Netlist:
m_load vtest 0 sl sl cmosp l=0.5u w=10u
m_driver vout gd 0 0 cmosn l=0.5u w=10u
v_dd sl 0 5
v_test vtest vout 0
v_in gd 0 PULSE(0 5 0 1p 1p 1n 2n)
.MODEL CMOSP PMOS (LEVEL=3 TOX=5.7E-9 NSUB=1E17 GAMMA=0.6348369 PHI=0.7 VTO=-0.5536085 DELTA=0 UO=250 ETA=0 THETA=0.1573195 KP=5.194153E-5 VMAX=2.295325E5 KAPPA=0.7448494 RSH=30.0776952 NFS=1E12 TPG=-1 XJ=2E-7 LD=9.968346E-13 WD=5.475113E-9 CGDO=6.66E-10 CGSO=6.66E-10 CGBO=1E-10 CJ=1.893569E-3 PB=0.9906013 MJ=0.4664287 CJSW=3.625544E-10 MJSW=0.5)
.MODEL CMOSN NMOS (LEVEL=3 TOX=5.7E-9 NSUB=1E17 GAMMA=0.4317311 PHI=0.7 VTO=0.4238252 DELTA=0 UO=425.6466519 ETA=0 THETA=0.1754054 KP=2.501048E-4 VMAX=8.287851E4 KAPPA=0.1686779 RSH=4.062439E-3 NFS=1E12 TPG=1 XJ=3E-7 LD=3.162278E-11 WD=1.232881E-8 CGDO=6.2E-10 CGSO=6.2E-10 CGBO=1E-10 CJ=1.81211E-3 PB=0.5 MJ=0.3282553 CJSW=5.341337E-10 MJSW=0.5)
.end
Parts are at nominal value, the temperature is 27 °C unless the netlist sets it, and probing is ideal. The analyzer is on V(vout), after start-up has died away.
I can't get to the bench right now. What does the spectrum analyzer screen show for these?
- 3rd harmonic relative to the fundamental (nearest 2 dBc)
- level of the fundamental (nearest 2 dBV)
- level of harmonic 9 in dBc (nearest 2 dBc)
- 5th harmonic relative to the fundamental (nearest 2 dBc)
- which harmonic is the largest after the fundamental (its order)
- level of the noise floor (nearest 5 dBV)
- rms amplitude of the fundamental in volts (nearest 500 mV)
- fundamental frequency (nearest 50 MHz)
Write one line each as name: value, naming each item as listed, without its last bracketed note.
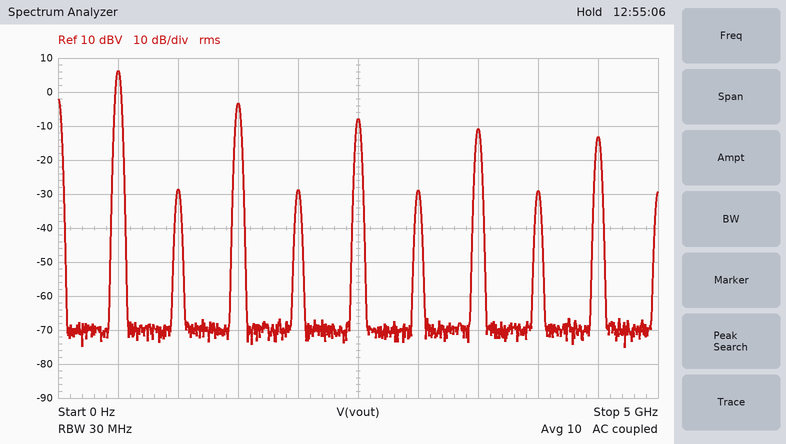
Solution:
3rd harmonic relative to the fundamental: -10 dBc
level of the fundamental: 6 dBV
level of harmonic 9 in dBc: -20 dBc
5th harmonic relative to the fundamental: -14 dBc
which harmonic is the largest after the fundamental: 3
level of the noise floor: -70 dBV
rms amplitude of the fundamental in volts: 2.0 V
fundamental frequency: 500 MHz
